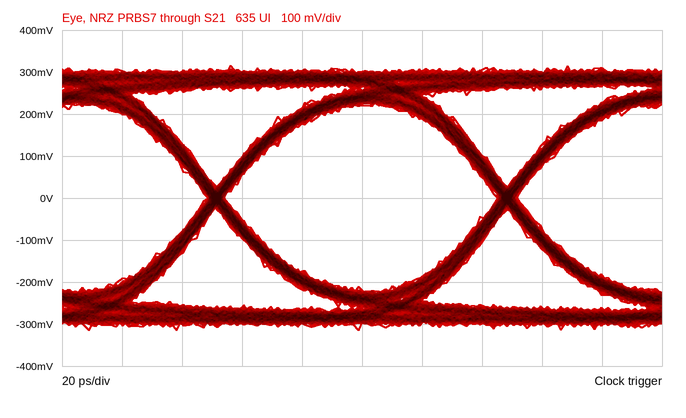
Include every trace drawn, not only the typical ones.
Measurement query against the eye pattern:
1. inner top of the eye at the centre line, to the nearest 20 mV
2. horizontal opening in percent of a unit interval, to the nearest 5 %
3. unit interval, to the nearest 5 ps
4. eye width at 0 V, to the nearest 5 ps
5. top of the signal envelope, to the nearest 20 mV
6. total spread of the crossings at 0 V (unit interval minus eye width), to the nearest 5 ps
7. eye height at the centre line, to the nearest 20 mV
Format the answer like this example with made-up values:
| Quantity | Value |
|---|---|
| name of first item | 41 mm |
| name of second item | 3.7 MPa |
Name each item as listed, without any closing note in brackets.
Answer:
| Quantity | Value |
|---|---|
| inner top of the eye at the centre line, to the nearest 20 mV | 220 mV |
| horizontal opening in percent of a unit interval, to the nearest 5 % | 95 % |
| unit interval, to the nearest 5 ps | 95 ps |
| eye width at 0 V, to the nearest 5 ps | 90 ps |
| top of the signal envelope, to the nearest 20 mV | 320 mV |
| total spread of the crossings at 0 V (unit interval minus eye width), to the nearest 5 ps | 5 ps |
| eye height at the centre line, to the nearest 20 mV | 440 mV |
